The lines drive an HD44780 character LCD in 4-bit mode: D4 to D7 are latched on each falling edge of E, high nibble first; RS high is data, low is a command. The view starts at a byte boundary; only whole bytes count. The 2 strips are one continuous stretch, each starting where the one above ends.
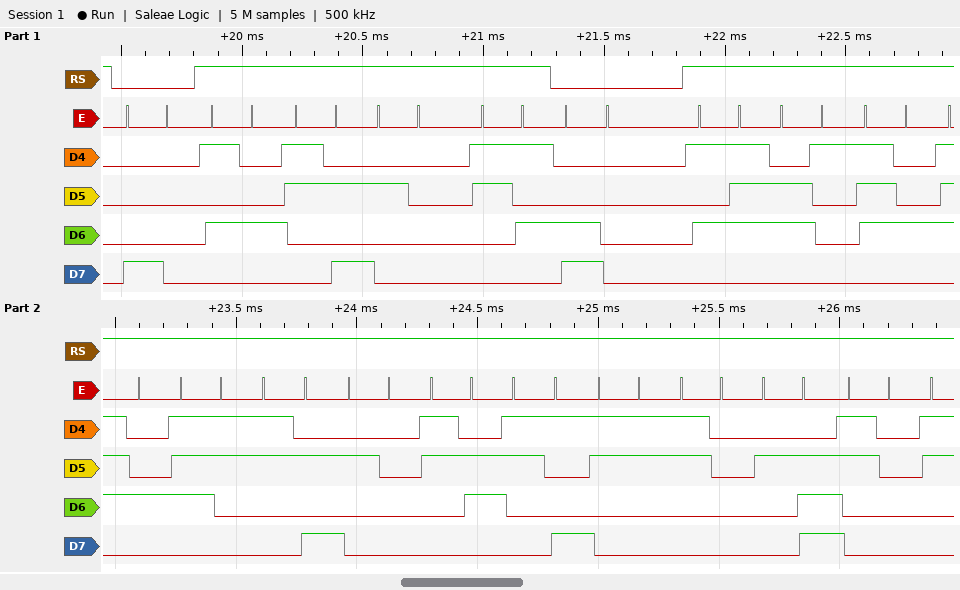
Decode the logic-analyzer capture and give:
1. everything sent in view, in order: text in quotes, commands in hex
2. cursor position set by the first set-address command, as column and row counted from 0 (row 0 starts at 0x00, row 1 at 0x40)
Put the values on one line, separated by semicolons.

0x80 "T: 5" 0xC0 "Watts: 6930.0"; column 0, row 0
